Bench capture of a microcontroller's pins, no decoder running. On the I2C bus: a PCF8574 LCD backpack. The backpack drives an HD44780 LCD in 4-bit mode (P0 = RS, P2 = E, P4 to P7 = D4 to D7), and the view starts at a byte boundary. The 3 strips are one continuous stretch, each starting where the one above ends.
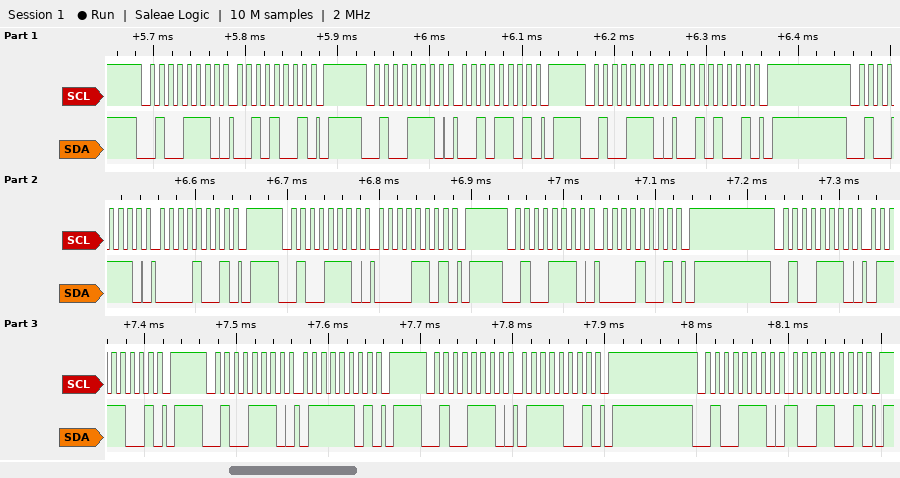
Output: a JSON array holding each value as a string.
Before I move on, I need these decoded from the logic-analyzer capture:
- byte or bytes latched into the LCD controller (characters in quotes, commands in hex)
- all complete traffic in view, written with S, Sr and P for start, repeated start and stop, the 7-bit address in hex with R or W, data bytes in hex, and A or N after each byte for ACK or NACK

["' '", "S 27W A 29 A P S 27W A 2D A P S 27W A 29 A P S 27W A 09 A P S 27W A 0D A P S 27W A 09 A P S 27W A 79 A P S 27W A 7D A P S 27W A 79 A P S 27W A 99 A P"]
